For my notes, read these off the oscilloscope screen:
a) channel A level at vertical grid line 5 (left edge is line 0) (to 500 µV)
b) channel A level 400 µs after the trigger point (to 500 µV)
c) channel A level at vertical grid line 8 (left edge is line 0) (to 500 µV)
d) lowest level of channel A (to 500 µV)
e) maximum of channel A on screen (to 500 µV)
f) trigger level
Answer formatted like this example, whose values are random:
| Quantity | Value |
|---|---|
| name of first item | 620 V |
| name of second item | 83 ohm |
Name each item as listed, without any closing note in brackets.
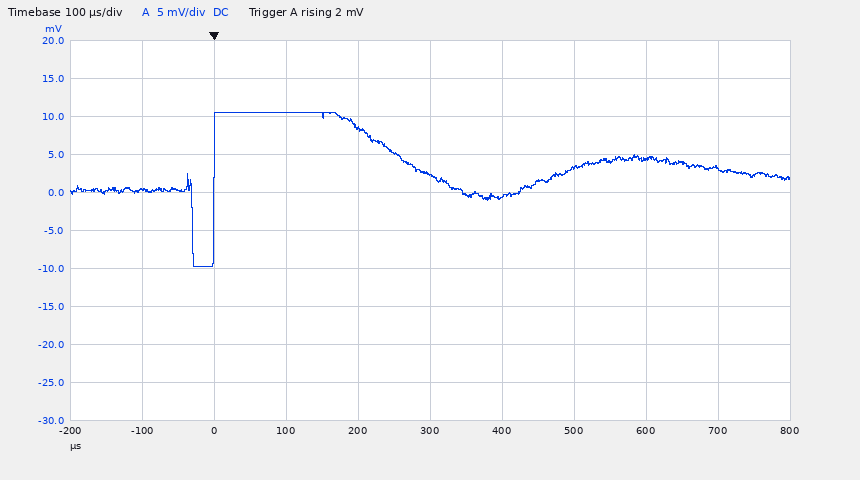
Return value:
| Quantity | Value |
|---|---|
| channel A level at vertical grid line 5 (left edge is line 0) | 2.5 mV |
| channel A level 400 µs after the trigger point | -500 µV |
| channel A level at vertical grid line 8 (left edge is line 0) | 4.5 mV |
| lowest level of channel A | -9.5 mV |
| maximum of channel A on screen | 10.5 mV |
| trigger level | 2 mV |
